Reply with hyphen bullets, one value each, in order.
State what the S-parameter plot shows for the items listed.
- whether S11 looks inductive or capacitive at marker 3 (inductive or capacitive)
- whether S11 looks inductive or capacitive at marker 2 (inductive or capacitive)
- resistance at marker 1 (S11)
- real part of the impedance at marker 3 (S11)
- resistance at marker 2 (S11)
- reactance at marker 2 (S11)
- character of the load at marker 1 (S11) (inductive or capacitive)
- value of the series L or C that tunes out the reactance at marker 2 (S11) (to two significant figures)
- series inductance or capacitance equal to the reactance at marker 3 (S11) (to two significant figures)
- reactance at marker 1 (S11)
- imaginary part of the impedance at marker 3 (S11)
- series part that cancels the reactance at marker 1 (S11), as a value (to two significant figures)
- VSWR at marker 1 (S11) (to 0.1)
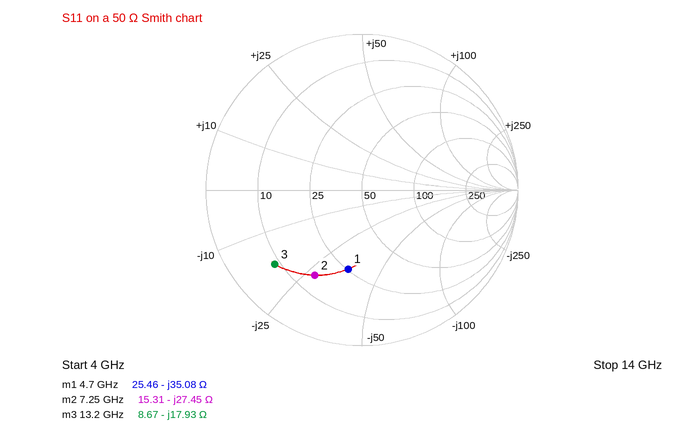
- capacitive
- capacitive
- 25.46 Ω
- 8.67 Ω
- 15.31 Ω
- -27.45 Ω
- capacitive
- 600 pH
- 670 fF
- -35.08 Ω
- -17.93 Ω
- 1.2 nH
- 3.1
